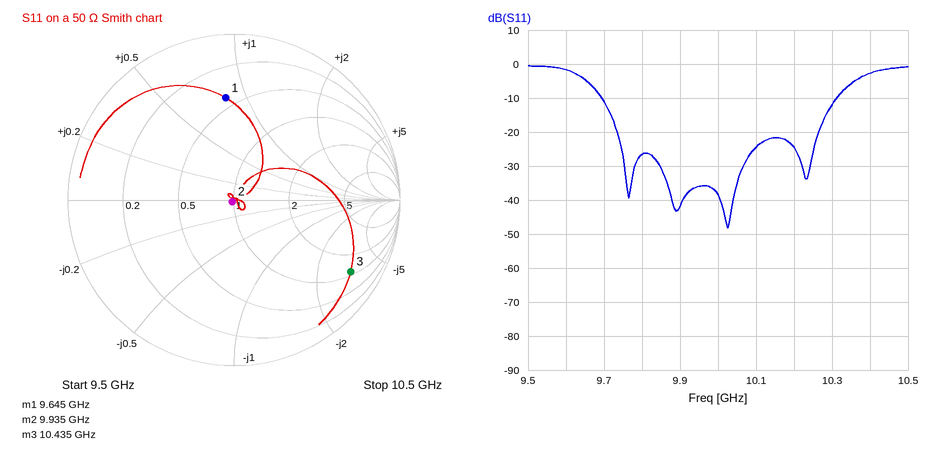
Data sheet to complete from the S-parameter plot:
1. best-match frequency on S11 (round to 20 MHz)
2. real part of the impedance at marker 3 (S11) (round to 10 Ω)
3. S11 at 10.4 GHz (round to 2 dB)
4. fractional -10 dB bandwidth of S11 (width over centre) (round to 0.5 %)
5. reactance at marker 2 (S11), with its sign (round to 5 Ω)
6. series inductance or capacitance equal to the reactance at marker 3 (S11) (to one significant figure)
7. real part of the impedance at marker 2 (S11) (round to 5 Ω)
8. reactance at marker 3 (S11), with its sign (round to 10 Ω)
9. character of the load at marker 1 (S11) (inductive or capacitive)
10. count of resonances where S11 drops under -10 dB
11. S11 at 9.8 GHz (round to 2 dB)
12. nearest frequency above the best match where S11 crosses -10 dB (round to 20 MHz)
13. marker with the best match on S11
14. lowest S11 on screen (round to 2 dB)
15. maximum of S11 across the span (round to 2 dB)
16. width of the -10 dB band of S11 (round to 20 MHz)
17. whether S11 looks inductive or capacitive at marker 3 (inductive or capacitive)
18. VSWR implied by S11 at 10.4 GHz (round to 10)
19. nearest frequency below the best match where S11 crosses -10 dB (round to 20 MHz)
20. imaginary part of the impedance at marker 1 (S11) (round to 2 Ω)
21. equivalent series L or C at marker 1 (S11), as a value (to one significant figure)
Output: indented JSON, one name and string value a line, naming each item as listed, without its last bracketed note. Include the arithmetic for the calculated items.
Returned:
{
  "best-match frequency on S11": "10.02 GHz",
  "real part of the impedance at marker 3 (S11)": "60 Ω",
  "S11 at 10.4 GHz": "-2 dB",
  "fractional -10 dB bandwidth of S11 (width over centre)": "620 MHz / 10.01 GHz ≈ 6.19 %, so 6.0 % to the nearest 0.5 %",
  "reactance at marker 2 (S11), with its sign": "0 Ω",
  "series inductance or capacitance equal to the reactance at marker 3 (S11)": "C = 1/(2π × 10.435 GHz × 160 Ω) ≈ 95.3 fF, so 100 fF to one significant figure",
  "real part of the impedance at marker 2 (S11)": "50 Ω",
  "reactance at marker 3 (S11), with its sign": "-160 Ω",
  "character of the load at marker 1 (S11)": "inductive",
  "count of resonances where S11 drops under -10 dB": "4",
  "S11 at 9.8 GHz": "-26 dB",
  "nearest frequency above the best match where S11 crosses -10 dB": "10.32 GHz",
  "marker with the best match on S11": "marker 2",
  "lowest S11 on screen": "-48 dB",
  "maximum of S11 across the span": "0 dB",
  "width of the -10 dB band of S11": "10.32 GHz − 9.70 GHz = 620 MHz",
  "whether S11 looks inductive or capacitive at marker 3": "capacitive",
  "VSWR implied by S11 at 10.4 GHz": "|Γ| = 10^(-2/20) = 0.7943; VSWR = (1 + 0.7943)/(1 − 0.7943) ≈ 8.72, so 10 to the nearest 10",
  "nearest frequency below the best match where S11 crosses -10 dB": "9.70 GHz",
  "imaginary part of the impedance at marker 1 (S11)": "+42 Ω",
  "equivalent series L or C at marker 1 (S11), as a value": "L = 42 Ω/(2π × 9.645 GHz) ≈ 693 pH, so 700 pH to one significant figure"
}
